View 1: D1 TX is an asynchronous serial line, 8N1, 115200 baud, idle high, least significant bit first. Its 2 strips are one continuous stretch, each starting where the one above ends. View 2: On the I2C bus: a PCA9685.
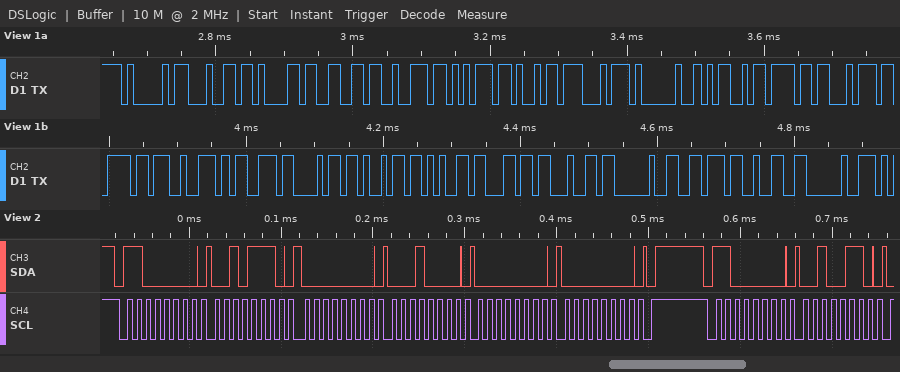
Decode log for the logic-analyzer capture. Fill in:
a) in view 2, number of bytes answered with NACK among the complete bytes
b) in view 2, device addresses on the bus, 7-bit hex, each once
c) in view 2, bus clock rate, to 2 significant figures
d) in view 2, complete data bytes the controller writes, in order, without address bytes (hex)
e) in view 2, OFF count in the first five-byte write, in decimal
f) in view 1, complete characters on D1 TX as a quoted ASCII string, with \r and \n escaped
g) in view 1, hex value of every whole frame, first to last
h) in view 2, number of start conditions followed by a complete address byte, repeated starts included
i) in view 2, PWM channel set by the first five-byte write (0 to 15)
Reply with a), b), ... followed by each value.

a) 0
b) 0x60
c) 100 kHz
d) 2E 00 10 00 00 26
e) 0
f) "Adafruit Motorshield v2 "
g) 41 64 61 66 72 75 69 74 20 4D 6F 74 6F 72 73 68 69 65 6C 64 20 76 32 20
h) 2
i) 10
